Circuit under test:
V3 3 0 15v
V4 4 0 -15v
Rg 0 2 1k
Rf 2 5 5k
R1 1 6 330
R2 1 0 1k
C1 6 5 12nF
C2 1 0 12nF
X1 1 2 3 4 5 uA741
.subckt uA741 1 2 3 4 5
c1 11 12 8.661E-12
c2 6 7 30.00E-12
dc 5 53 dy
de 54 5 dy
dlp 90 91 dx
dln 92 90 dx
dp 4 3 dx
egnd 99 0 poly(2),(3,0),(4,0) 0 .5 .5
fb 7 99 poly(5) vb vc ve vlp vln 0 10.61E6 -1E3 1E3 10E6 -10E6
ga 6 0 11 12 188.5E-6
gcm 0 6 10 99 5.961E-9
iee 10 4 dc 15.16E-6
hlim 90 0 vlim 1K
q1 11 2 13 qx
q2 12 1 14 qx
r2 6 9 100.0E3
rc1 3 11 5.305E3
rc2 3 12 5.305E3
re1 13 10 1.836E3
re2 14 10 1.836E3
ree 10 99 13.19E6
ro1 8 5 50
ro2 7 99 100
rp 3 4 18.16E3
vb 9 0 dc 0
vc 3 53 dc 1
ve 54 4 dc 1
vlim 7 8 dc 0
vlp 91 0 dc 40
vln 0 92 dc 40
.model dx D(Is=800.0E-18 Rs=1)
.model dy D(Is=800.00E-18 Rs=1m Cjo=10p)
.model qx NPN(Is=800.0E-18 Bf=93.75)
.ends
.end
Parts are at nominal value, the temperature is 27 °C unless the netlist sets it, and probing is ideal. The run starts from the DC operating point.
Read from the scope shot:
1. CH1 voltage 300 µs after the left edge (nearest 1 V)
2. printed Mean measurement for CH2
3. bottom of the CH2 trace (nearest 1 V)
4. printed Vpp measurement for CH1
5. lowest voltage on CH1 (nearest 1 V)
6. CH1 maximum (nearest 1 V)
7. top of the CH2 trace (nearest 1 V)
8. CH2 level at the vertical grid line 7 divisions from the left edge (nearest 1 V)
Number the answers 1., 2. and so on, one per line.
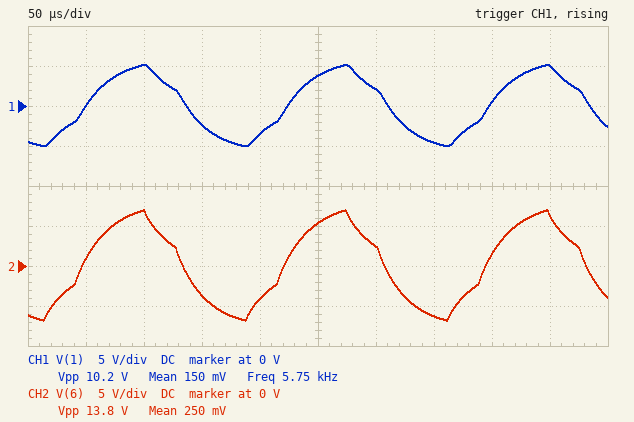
1. 2 V
2. 250 mV
3. -7 V
4. 10.2 V
5. -5 V
6. 5 V
7. 7 V
8. -6 V
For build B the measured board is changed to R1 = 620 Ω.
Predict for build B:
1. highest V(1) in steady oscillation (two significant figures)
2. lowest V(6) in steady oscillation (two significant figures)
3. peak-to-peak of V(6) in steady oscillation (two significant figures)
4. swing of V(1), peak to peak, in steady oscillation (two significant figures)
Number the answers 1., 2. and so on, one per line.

1. 4.9 V
2. -8.1 V
3. 16 V
4. 9.8 V
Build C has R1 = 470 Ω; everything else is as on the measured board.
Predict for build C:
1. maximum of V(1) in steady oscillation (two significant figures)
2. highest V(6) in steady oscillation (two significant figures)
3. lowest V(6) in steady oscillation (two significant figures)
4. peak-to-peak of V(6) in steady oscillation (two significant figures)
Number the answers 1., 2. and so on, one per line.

1. 5.0 V
2. 7.6 V
3. -7.5 V
4. 15 V
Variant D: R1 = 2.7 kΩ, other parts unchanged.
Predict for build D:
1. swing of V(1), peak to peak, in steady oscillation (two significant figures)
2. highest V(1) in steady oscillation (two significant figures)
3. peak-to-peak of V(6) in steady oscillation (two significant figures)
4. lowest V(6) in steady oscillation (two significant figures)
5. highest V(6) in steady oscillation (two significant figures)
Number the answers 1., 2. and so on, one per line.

1. 6.7 V
2. 3.3 V
3. 27 V
4. -14 V
5. 14 V
